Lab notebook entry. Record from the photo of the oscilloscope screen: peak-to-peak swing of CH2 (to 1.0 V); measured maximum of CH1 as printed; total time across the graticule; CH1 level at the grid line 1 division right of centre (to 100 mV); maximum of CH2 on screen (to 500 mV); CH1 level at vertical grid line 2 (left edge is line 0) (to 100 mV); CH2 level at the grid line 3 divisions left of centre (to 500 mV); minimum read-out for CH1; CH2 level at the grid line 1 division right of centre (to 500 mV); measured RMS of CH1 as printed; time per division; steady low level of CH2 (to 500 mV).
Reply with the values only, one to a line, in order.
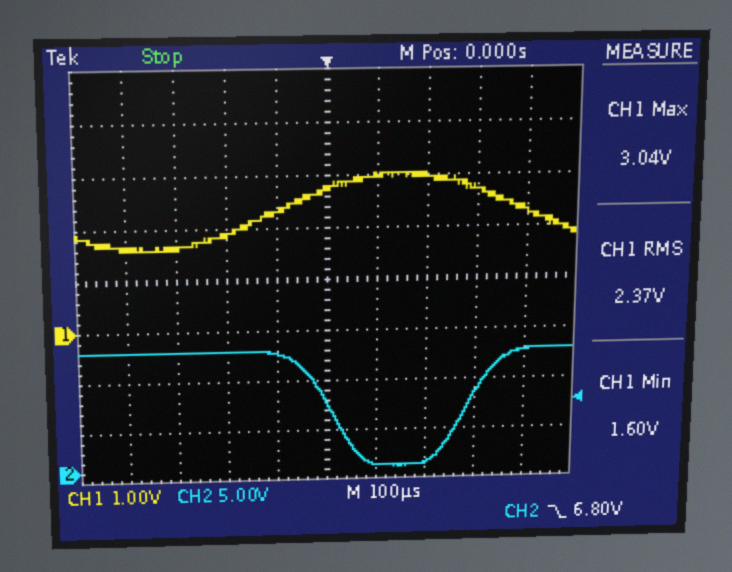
12.0 V
3.04 V
1 ms
3.0 V
12.0 V
1.6 V
12.0 V
1.60 V
500 mV
2.37 V
100 µs
500 mV
